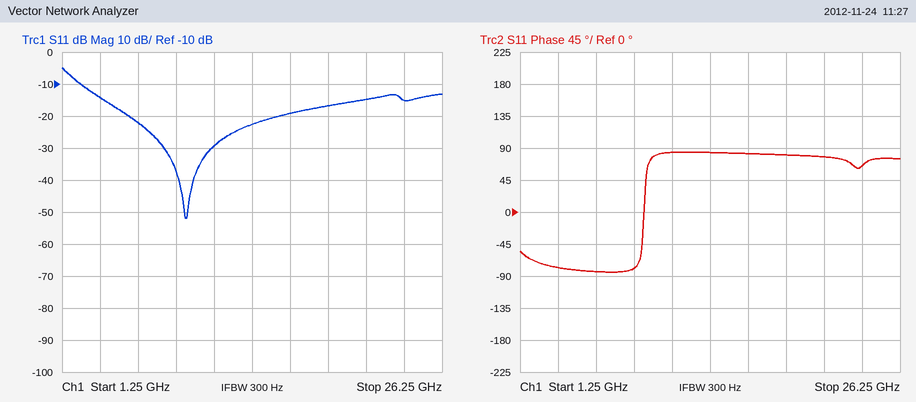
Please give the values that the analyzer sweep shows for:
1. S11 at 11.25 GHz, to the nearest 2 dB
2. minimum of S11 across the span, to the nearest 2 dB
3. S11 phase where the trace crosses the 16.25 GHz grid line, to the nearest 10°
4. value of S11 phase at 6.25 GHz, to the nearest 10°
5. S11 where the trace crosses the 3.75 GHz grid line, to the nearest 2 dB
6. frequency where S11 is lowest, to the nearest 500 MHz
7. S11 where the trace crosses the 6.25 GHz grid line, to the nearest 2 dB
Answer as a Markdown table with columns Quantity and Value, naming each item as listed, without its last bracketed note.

| Quantity | Value |
|---|---|
| S11 at 11.25 GHz, to the nearest 2 dB | -30 dB |
| minimum of S11 across the span, to the nearest 2 dB | -52 dB |
| S11 phase where the trace crosses the 16.25 GHz grid line, to the nearest 10° | 80° |
| value of S11 phase at 6.25 GHz, to the nearest 10° | -80° |
| S11 where the trace crosses the 3.75 GHz grid line, to the nearest 2 dB | -14 dB |
| frequency where S11 is lowest, to the nearest 500 MHz | 9.5 GHz |
| S11 where the trace crosses the 6.25 GHz grid line, to the nearest 2 dB | -22 dB |
